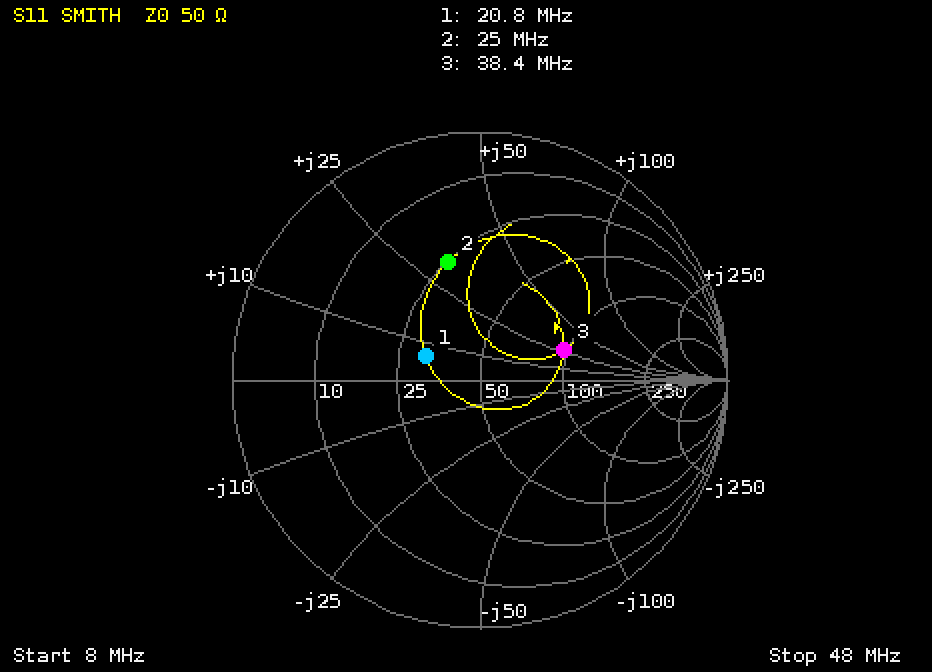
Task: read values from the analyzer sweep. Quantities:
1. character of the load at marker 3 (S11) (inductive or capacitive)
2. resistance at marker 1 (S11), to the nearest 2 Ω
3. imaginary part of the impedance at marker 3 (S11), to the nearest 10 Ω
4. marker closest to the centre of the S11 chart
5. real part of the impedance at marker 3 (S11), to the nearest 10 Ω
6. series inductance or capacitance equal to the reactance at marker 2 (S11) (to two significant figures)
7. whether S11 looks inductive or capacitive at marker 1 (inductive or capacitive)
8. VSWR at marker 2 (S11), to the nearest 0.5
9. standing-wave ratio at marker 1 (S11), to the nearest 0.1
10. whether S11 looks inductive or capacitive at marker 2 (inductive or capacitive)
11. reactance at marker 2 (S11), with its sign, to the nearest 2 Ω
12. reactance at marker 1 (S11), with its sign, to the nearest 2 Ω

inductive
32 Ω
+30 Ω
marker 1
100 Ω
200 nH
inductive
3.0
1.6
inductive
+32 Ω
+6 Ω
